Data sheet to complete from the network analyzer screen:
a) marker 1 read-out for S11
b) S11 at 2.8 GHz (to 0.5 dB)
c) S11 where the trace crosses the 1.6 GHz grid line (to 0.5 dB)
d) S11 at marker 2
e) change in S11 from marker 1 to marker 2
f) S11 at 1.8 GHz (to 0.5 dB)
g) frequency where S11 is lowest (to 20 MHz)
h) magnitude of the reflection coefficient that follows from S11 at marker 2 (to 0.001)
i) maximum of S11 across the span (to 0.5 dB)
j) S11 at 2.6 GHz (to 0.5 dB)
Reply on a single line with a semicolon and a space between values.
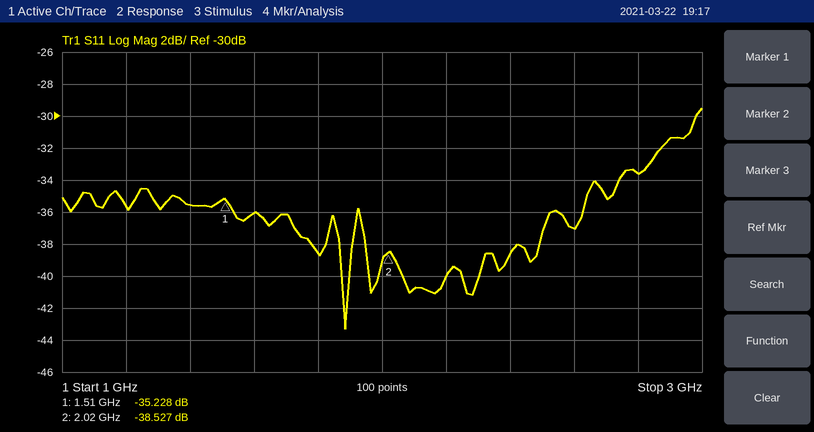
-35.228 dB; -33.5 dB; -36.0 dB; -38.527 dB; -3.299 dB; -38.5 dB; 1.88 GHz; 0.012; -29.5 dB; -37.0 dB
